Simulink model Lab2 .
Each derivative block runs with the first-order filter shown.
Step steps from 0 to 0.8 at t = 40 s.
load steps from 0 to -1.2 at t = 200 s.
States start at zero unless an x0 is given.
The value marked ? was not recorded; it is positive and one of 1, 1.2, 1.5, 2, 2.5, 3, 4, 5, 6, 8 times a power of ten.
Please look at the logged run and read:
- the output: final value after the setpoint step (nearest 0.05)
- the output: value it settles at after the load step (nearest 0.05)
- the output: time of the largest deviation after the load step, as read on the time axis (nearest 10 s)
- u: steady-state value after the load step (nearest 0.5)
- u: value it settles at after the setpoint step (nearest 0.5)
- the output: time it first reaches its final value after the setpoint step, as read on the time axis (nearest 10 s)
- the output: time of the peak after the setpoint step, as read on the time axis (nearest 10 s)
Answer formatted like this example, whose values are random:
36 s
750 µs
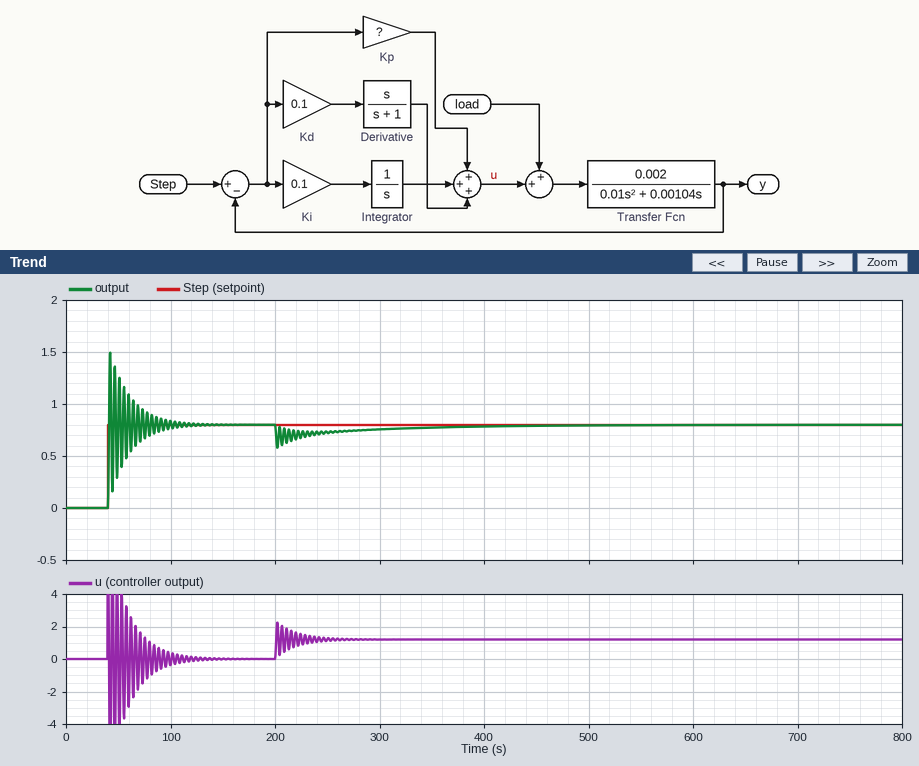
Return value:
0.80
0.80
200 s
1.0
0.0
40 s
40 s
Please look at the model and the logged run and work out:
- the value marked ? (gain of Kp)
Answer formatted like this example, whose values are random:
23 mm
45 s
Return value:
10
